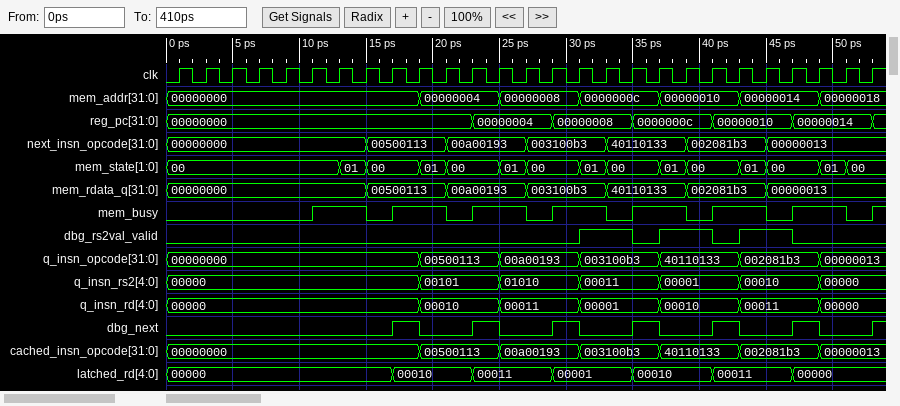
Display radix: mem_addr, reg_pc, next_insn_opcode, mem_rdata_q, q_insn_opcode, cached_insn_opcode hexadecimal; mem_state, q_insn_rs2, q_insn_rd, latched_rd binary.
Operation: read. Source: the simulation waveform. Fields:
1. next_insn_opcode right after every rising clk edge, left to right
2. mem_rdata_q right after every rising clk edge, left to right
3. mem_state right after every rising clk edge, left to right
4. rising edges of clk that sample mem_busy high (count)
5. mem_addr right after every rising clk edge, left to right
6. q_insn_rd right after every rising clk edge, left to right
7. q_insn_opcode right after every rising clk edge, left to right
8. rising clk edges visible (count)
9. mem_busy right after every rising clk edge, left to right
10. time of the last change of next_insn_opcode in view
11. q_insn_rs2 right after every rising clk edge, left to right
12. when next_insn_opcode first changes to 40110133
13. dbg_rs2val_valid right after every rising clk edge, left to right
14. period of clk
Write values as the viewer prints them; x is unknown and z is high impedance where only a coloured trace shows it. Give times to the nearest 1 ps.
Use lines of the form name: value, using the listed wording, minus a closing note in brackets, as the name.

next_insn_opcode right after every rising clk edge, left to right: 00000000, 00000000, 00000000, 00000000, 00000000, 00000000, 00000000, 00500113, 00500113, 00500113, 00a00193, 00a00193, 00a00193, 003100b3, 003100b3, 003100b3, 40110133, 40110133, 40110133, 002081b3, 002081b3, 002081b3, 00000013, 00000013, 00000013, 00000013, 00000013
mem_rdata_q right after every rising clk edge, left to right: 00000000, 00000000, 00000000, 00000000, 00000000, 00000000, 00000000, 00500113, 00500113, 00500113, 00a00193, 00a00193, 00a00193, 003100b3, 003100b3, 003100b3, 40110133, 40110133, 40110133, 002081b3, 002081b3, 002081b3, 00000013, 00000013, 00000013, 00000013, 00000013
mem_state right after every rising clk edge, left to right: 00, 00, 00, 00, 00, 00, 01, 00, 00, 01, 00, 00, 01, 00, 00, 01, 00, 00, 01, 00, 00, 01, 00, 00, 01, 00, 00
rising edges of clk that sample mem_busy high: 14
mem_addr right after every rising clk edge, left to right: 00000000, 00000000, 00000000, 00000000, 00000000, 00000000, 00000000, 00000000, 00000000, 00000004, 00000004, 00000004, 00000008, 00000008, 00000008, 0000000c, 0000000c, 0000000c, 00000010, 00000010, 00000010, 00000014, 00000014, 00000014, 00000018, 00000018, 00000018
q_insn_rd right after every rising clk edge, left to right: 00000, 00000, 00000, 00000, 00000, 00000, 00000, 00000, 00000, 00010, 00010, 00010, 00011, 00011, 00011, 00001, 00001, 00001, 00010, 00010, 00010, 00011, 00011, 00011, 00000, 00000, 00000
q_insn_opcode right after every rising clk edge, left to right: 00000000, 00000000, 00000000, 00000000, 00000000, 00000000, 00000000, 00000000, 00000000, 00500113, 00500113, 00500113, 00a00193, 00a00193, 00a00193, 003100b3, 003100b3, 003100b3, 40110133, 40110133, 40110133, 002081b3, 002081b3, 002081b3, 00000013, 00000013, 00000013
rising clk edges visible: 27
mem_busy right after every rising clk edge, left to right: 0 0 0 0 0 1 1 0 1 1 0 1 1 0 1 1 0 1 1 0 1 1 0 1 1 0 1
time of the last change of next_insn_opcode in view: 45 ps
q_insn_rs2 right after every rising clk edge, left to right: 00000, 00000, 00000, 00000, 00000, 00000, 00000, 00000, 00000, 00101, 00101, 00101, 01010, 01010, 01010, 00011, 00011, 00011, 00001, 00001, 00001, 00010, 00010, 00010, 00000, 00000, 00000
when next_insn_opcode first changes to 40110133: 33 ps
dbg_rs2val_valid right after every rising clk edge, left to right: 0 0 0 0 0 0 0 0 0 0 0 0 0 0 0 1 1 0 1 1 0 1 1 0 0 0 0
period of clk: 2 ps
